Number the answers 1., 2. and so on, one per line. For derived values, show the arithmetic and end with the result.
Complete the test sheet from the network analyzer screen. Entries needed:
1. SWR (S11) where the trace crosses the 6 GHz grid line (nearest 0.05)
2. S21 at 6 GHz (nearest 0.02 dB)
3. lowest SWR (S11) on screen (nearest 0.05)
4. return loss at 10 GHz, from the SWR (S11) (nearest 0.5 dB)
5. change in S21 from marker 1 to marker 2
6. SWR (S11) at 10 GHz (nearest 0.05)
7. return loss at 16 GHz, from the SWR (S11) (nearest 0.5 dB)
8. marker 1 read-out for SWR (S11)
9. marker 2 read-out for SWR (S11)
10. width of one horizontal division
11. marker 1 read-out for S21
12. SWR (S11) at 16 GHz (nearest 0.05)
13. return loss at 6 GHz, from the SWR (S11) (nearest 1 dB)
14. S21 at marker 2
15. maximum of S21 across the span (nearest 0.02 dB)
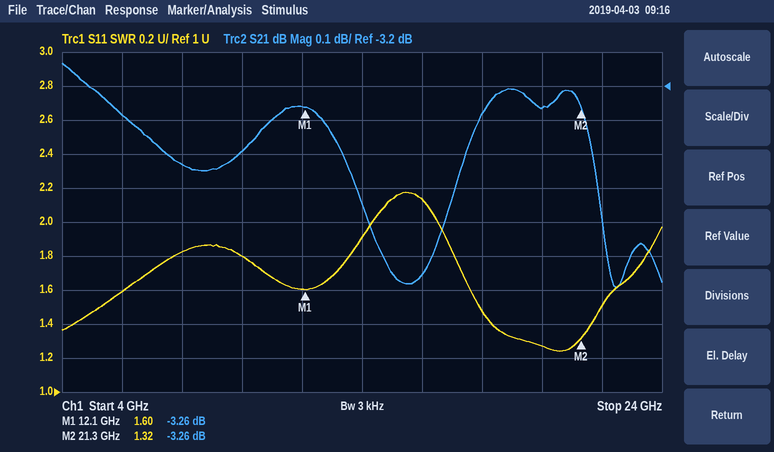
1. 1.60
2. -3.28 dB
3. 1.25
4. −20 log10((1.8 − 1)/(1.8 + 1)) ≈ 10.9 dB, so 11.0 dB to the nearest 0.5 dB
5. -3.26 − (-3.26) = 0.00 dB
6. 1.80
7. −20 log10((2.15 − 1)/(2.15 + 1)) ≈ 8.75 dB, so 9.0 dB to the nearest 0.5 dB
8. 1.60
9. 1.32
10. 2 GHz
11. -3.26 dB
12. 2.15
13. −20 log10((1.6 − 1)/(1.6 + 1)) ≈ 13 dB
14. -3.26 dB
15. -3.14 dB
